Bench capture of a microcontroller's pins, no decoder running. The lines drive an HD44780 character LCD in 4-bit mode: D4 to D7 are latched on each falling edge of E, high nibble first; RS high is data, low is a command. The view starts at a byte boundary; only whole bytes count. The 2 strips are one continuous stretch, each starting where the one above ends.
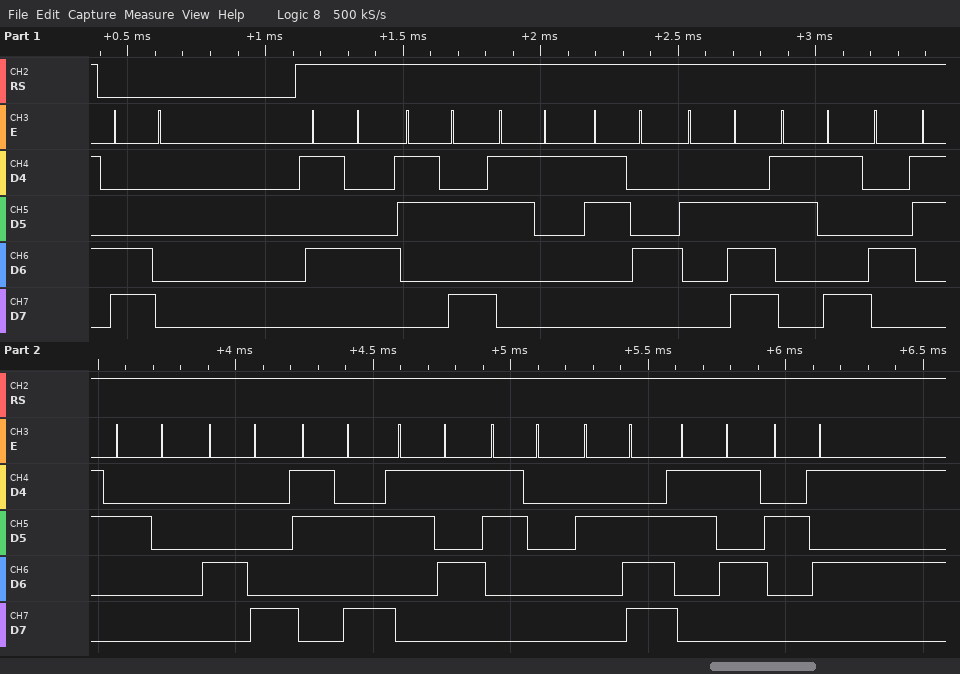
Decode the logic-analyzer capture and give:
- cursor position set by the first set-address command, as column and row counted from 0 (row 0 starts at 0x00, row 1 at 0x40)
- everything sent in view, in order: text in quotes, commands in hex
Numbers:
column 0, row 1
0xC0 "T:14.9C H:50.5%"
